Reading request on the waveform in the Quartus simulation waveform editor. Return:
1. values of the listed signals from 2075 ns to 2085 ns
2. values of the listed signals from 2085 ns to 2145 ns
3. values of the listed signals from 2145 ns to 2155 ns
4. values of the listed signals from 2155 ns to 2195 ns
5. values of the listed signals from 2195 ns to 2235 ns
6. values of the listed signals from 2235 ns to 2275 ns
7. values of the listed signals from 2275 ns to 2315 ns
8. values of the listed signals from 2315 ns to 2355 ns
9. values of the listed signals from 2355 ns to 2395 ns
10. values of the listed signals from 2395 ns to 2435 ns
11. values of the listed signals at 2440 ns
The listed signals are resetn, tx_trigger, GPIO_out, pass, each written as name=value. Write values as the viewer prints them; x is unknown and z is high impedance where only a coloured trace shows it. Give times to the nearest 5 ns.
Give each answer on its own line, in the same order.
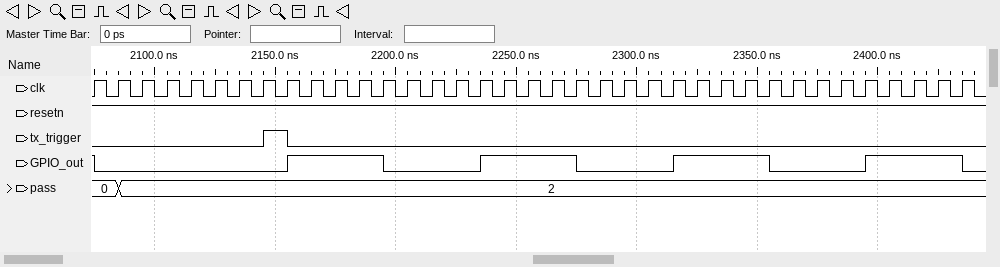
resetn=1, tx_trigger=0, GPIO_out=0, pass=0
resetn=1, tx_trigger=0, GPIO_out=0, pass=2
resetn=1, tx_trigger=1, GPIO_out=0, pass=2
resetn=1, tx_trigger=0, GPIO_out=1, pass=2
resetn=1, tx_trigger=0, GPIO_out=0, pass=2
resetn=1, tx_trigger=0, GPIO_out=1, pass=2
resetn=1, tx_trigger=0, GPIO_out=0, pass=2
resetn=1, tx_trigger=0, GPIO_out=1, pass=2
resetn=1, tx_trigger=0, GPIO_out=0, pass=2
resetn=1, tx_trigger=0, GPIO_out=1, pass=2
resetn=1, tx_trigger=0, GPIO_out=0, pass=2
